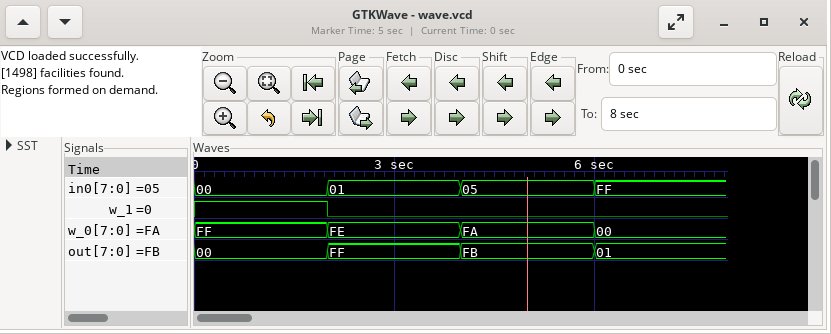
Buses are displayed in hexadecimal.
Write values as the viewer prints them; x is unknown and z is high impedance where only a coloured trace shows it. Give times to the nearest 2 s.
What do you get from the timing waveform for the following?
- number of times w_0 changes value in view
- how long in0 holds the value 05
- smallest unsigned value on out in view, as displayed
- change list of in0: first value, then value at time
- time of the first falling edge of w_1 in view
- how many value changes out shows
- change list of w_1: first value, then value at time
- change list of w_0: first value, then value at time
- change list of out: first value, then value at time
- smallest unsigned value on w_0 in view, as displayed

3
2 s
00
00, 01 at 2 s, 05 at 4 s, FF at 6 s
2 s
3
1, 0 at 2 s
FF, FE at 2 s, FA at 4 s, 00 at 6 s
00, FF at 2 s, FB at 4 s, 01 at 6 s
00
